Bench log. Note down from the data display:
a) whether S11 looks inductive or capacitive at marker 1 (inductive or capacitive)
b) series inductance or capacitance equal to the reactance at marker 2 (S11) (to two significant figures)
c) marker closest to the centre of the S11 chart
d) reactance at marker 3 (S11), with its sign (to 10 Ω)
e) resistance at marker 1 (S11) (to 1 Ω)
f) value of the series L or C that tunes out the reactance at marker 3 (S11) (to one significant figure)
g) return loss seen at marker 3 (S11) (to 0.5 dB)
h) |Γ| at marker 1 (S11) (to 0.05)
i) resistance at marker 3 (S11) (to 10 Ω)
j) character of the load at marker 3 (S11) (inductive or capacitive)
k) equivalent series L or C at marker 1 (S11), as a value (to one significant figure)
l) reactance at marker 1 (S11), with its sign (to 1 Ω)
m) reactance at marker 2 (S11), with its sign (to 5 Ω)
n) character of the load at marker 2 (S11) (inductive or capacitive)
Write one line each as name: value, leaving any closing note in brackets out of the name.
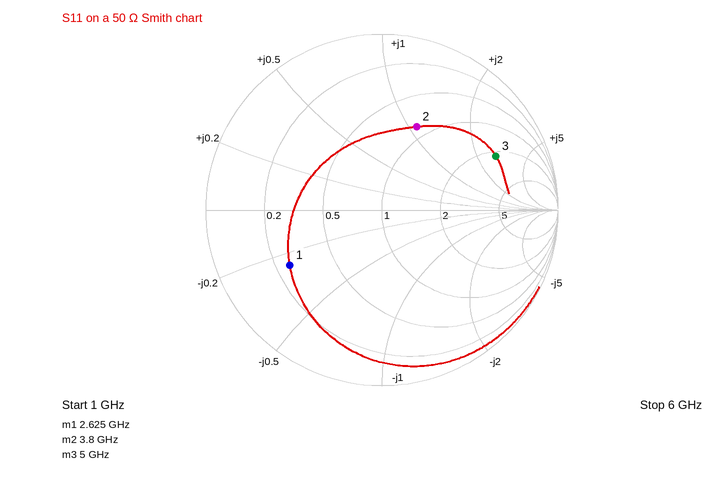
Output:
whether S11 looks inductive or capacitive at marker 1: capacitive
series inductance or capacitance equal to the reactance at marker 2 (S11): 2.3 nH
marker closest to the centre of the S11 chart: marker 2
reactance at marker 3 (S11), with its sign: +140 Ω
resistance at marker 1 (S11): 13 Ω
value of the series L or C that tunes out the reactance at marker 3 (S11): 200 fF
return loss seen at marker 3 (S11): 3.0 dB
|Γ| at marker 1 (S11): 0.60
resistance at marker 3 (S11): 110 Ω
character of the load at marker 3 (S11): inductive
equivalent series L or C at marker 1 (S11), as a value: 5 pF
reactance at marker 1 (S11), with its sign: -13 Ω
reactance at marker 2 (S11), with its sign: +55 Ω
character of the load at marker 2 (S11): inductive
